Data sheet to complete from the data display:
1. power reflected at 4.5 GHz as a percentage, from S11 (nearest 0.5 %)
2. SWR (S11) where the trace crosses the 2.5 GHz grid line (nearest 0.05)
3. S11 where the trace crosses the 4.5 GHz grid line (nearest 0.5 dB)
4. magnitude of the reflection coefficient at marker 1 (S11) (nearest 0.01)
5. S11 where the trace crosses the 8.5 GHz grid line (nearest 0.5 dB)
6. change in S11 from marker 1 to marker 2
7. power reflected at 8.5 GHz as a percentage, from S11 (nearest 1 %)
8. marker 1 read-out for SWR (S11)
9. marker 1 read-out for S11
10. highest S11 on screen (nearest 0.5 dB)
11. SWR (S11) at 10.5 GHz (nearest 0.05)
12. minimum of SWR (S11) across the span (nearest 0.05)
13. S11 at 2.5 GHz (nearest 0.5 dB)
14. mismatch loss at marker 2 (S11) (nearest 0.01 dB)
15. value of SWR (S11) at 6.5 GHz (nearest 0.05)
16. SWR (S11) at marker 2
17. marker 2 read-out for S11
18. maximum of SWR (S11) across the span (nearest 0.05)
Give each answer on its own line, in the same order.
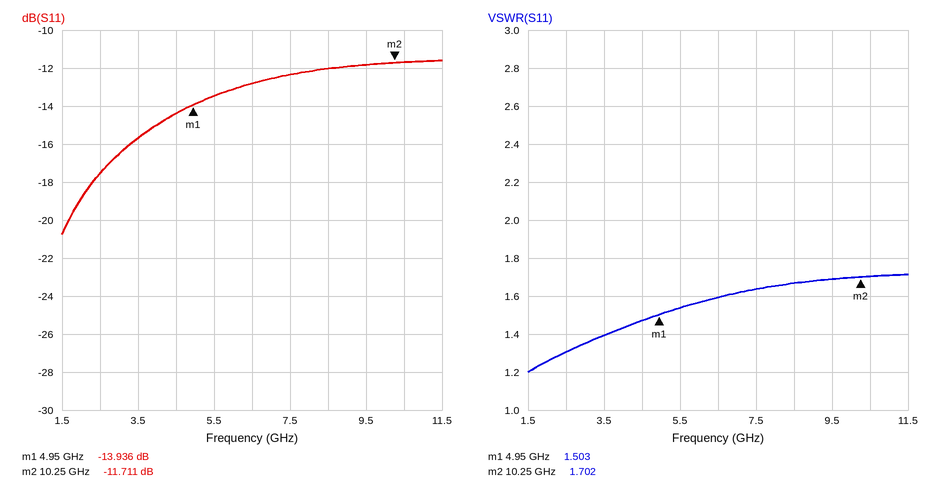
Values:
3.5 %
1.30
-14.5 dB
0.20
-12.0 dB
2.225 dB
6 %
1.503
-13.936 dB
-11.5 dB
1.70
1.20
-17.5 dB
0.30 dB
1.60
1.702
-11.711 dB
1.70
